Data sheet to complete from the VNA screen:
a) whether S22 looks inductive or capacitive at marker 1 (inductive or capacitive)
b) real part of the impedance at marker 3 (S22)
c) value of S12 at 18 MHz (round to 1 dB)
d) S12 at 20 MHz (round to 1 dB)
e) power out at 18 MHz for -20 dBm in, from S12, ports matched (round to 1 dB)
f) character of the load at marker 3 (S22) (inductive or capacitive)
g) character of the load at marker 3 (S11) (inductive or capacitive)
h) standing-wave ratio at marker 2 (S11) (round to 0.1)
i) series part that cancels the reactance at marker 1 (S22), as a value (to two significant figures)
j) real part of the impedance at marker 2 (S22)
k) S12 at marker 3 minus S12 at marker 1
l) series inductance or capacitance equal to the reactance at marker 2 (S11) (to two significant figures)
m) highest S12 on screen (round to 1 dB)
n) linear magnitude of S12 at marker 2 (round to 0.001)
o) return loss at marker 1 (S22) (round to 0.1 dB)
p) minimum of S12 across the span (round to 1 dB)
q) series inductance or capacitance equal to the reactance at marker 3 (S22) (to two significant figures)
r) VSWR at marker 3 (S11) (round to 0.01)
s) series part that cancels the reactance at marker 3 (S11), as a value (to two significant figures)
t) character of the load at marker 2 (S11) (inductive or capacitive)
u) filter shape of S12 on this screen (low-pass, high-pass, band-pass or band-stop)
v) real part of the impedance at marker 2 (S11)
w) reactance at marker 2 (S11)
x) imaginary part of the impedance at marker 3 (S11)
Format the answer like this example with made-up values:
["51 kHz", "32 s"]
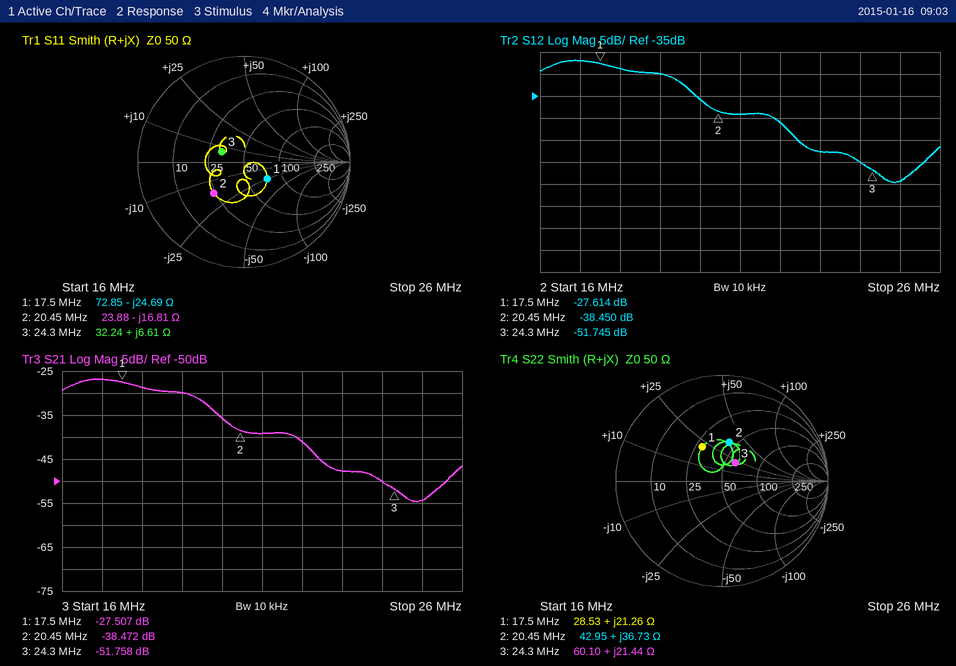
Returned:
["inductive", "60.10 Ω", "-29 dB", "-36 dB", "-49 dBm", "inductive", "inductive", "2.4", "430 pF", "42.95 Ω", "-24.131 dB", "460 pF", "-27 dB", "0.012", "8.6 dB", "-55 dB", "140 nH", "1.60", "990 pF", "capacitive", "low-pass", "23.88 Ω", "-16.81 Ω", "+6.61 Ω"]
